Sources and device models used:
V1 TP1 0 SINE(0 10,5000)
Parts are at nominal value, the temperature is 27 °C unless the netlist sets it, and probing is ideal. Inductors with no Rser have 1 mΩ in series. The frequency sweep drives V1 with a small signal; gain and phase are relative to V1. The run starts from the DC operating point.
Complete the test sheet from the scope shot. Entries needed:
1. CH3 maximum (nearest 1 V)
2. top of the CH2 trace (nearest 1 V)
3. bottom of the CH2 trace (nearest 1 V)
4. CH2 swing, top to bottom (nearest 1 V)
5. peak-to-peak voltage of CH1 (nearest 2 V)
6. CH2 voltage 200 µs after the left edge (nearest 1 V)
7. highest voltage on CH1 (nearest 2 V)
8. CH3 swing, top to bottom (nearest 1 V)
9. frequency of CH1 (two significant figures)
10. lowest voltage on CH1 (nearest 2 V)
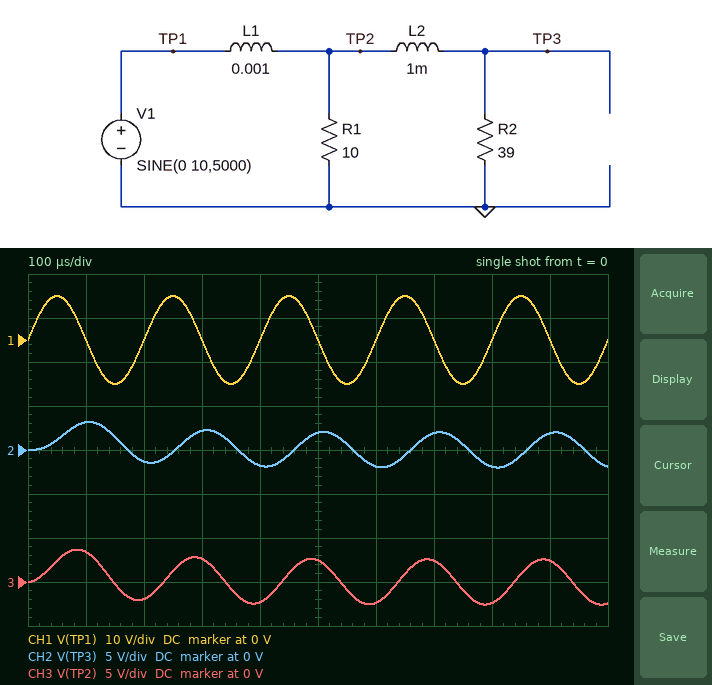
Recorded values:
4 V
3 V
-2 V
5 V
20 V
-1 V
10 V
6 V
5.0 kHz
-10 V
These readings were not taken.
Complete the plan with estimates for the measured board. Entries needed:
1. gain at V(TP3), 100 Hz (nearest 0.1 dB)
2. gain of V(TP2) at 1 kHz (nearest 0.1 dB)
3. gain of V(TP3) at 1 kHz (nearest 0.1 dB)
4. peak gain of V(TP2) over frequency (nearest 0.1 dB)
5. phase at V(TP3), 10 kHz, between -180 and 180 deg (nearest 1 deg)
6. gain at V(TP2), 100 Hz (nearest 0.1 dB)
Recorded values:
0 dB
-2.2 dB
-2.3 dB
0 dB
-134 deg
0 dB
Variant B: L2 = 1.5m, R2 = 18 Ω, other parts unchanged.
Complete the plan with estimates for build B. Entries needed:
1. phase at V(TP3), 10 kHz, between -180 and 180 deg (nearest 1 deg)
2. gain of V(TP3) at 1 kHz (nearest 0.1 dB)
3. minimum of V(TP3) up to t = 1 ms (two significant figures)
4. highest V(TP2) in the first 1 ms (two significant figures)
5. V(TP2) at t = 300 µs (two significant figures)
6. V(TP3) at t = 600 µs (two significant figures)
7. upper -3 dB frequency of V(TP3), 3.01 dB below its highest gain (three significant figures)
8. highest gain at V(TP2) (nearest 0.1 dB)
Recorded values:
-155 deg
-4.3 dB
-930 mV
3.6 V
2.7 V
-600 mV
776 Hz
0 dB
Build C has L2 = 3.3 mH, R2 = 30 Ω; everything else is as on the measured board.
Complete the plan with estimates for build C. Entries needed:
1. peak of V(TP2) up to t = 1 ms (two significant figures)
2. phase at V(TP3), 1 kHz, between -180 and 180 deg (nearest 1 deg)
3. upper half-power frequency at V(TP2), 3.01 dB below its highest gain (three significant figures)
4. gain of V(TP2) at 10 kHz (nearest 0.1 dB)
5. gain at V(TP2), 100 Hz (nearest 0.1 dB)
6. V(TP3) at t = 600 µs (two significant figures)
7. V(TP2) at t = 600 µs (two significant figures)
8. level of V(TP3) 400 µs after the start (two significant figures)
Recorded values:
3.9 V
-70 deg
1.15 kHz
-16.2 dB
0 dB
-400 mV
-2.6 V
-210 mV
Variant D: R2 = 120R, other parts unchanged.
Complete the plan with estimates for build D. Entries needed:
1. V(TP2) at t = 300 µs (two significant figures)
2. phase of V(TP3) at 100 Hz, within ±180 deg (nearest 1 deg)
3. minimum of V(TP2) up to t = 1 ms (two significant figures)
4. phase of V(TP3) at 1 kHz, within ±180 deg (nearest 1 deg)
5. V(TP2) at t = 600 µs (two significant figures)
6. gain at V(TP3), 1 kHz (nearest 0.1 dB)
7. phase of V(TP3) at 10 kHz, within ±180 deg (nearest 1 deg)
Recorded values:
2.9 V
-4 deg
-2.8 V
-37 deg
-2.7 V
-1.7 dB
-107 deg
